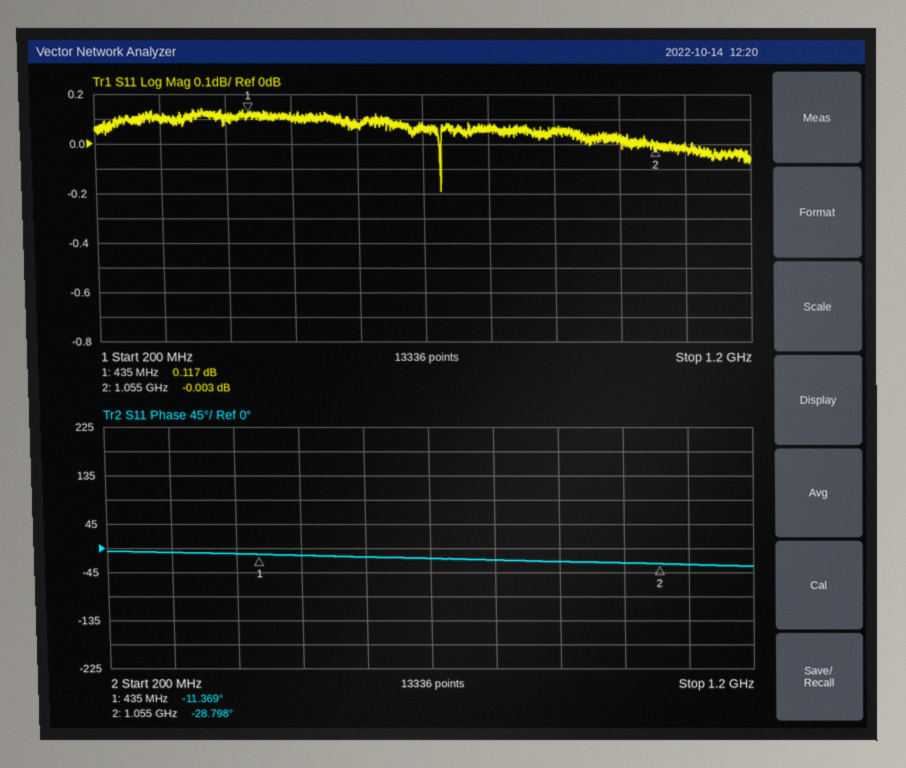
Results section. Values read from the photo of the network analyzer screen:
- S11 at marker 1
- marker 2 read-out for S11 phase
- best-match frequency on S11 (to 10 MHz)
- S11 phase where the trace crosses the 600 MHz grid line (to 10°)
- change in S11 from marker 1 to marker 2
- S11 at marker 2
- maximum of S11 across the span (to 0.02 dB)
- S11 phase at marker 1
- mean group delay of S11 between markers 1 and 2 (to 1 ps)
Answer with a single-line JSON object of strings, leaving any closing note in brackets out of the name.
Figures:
{"S11 at marker 1": "0.117 dB", "marker 2 read-out for S11 phase": "-28.798°", "best-match frequency on S11": "730 MHz", "S11 phase where the trace crosses the 600 MHz grid line": "-20°", "change in S11 from marker 1 to marker 2": "-0.120 dB", "S11 at marker 2": "-0.003 dB", "maximum of S11 across the span": "0.14 dB", "S11 phase at marker 1": "-11.369°", "mean group delay of S11 between markers 1 and 2": "78 ps"}
